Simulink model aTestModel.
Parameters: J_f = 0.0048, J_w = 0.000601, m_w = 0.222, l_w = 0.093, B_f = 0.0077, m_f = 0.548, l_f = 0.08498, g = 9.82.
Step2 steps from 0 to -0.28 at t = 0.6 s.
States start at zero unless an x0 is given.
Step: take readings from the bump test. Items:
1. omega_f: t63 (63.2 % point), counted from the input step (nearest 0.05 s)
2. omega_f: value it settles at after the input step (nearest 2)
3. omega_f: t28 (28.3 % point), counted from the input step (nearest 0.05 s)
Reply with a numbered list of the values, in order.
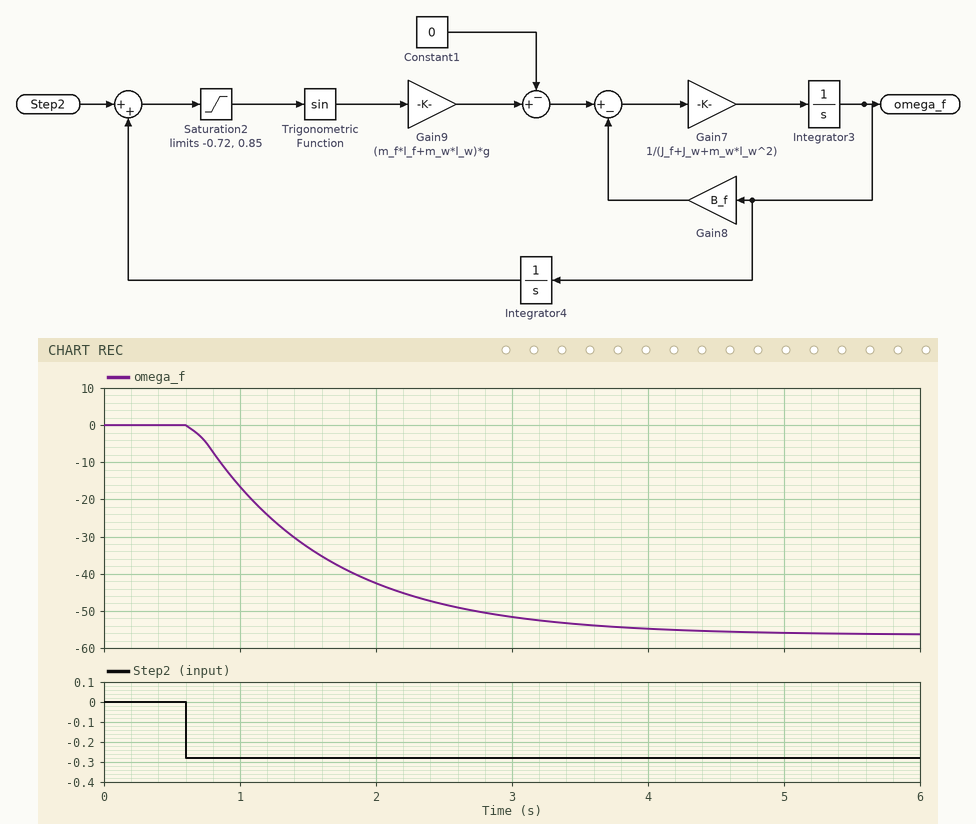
1. 1.00 s
2. -56
3. 0.40 s
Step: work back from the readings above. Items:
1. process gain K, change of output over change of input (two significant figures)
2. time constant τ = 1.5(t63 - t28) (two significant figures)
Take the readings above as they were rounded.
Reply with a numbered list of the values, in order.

1. 200
2. 0.90 s
